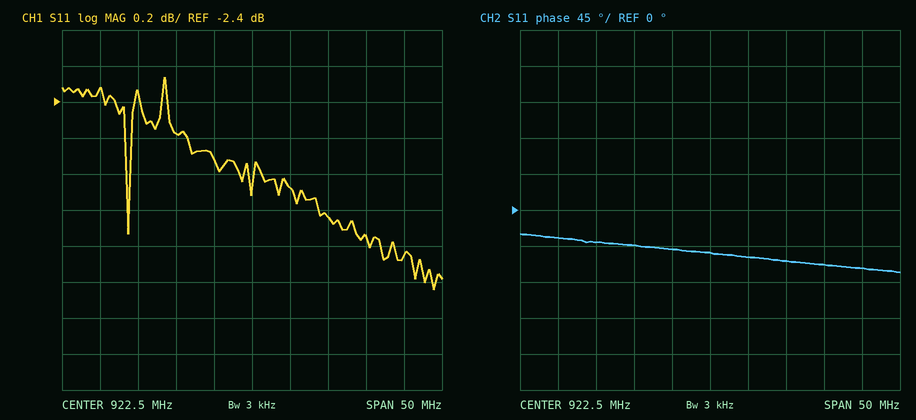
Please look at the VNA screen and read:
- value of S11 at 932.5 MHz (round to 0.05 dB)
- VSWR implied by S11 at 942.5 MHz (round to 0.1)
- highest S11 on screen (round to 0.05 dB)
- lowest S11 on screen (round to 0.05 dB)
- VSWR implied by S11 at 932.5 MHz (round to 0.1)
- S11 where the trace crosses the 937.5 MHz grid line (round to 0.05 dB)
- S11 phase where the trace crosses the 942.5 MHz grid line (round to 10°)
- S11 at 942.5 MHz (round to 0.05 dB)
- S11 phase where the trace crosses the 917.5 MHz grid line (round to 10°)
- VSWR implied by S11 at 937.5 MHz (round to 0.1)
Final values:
-3.05 dB
5.4
-2.25 dB
-3.45 dB
5.8
-3.15 dB
-70°
-3.25 dB
-50°
5.6
